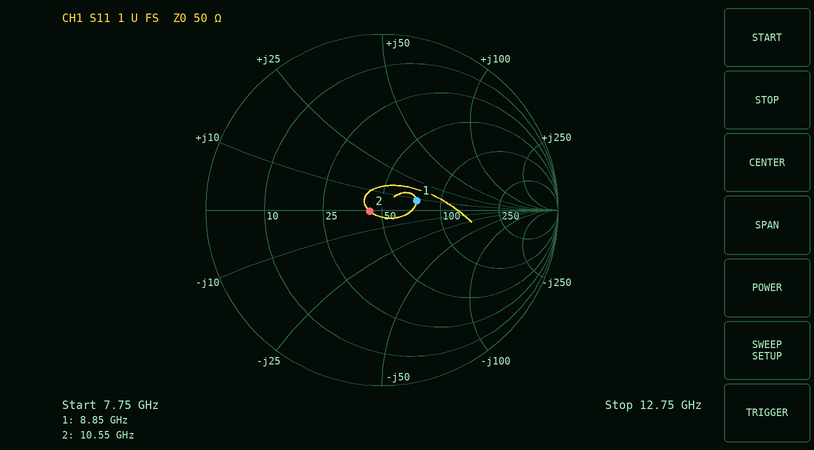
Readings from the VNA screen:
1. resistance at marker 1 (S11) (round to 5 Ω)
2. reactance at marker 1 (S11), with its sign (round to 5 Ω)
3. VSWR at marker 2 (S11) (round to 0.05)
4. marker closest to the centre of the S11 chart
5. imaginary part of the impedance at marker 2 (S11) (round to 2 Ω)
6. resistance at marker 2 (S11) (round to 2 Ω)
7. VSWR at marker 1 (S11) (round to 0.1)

75 Ω
+10 Ω
1.15
marker 2
0 Ω
44 Ω
1.5
